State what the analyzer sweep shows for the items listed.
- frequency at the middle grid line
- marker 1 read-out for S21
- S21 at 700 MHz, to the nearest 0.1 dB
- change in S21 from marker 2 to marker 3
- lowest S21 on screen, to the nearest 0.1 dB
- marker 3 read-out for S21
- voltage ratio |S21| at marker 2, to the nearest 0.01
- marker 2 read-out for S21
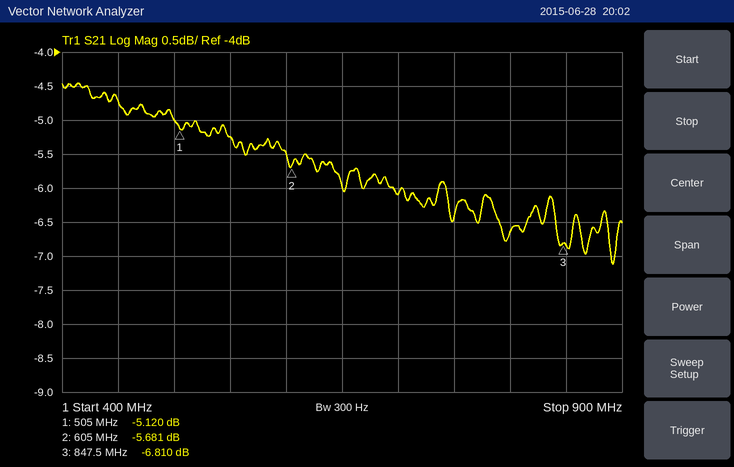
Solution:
650 MHz
-5.120 dB
-6.1 dB
-1.129 dB
-7.1 dB
-6.810 dB
0.52
-5.681 dB
